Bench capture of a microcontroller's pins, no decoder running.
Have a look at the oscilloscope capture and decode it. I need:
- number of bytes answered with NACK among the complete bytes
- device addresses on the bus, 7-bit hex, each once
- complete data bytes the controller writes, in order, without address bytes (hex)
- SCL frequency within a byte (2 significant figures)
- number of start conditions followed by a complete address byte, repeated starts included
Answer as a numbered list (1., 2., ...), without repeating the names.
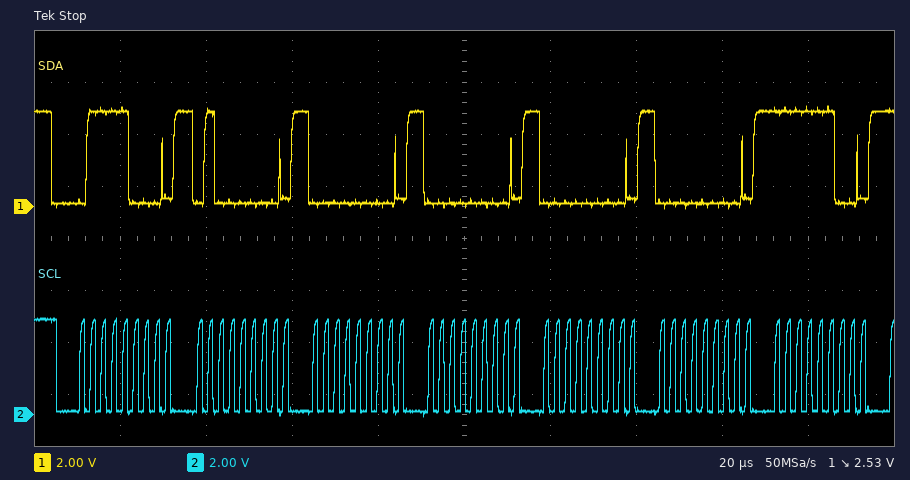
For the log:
1. 0
2. 0x3C
3. 40 00 00 00 00 FC
4. 400 kHz
5. 1
